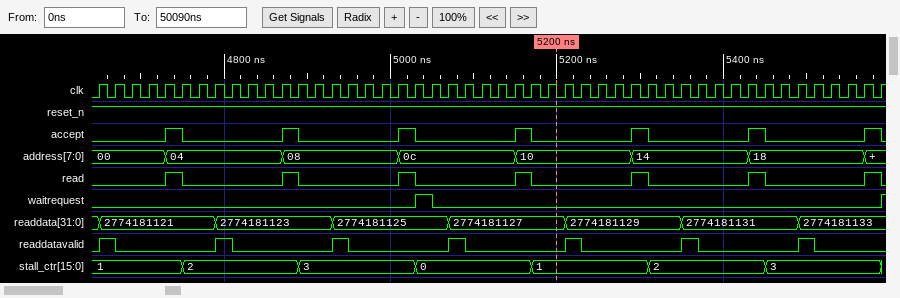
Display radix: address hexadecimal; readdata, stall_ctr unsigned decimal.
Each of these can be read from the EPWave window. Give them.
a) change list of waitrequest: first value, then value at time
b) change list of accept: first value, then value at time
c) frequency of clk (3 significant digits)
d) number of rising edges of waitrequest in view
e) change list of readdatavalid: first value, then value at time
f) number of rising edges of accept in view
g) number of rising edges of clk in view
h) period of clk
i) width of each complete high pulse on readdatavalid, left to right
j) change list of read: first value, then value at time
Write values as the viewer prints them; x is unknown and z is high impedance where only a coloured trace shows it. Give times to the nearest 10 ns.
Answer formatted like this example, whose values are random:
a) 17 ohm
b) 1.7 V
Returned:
a) 0, 1 at 5030 ns, 0 at 5050 ns, 1 at 5590 ns
b) 0, 1 at 4730 ns, 0 at 4750 ns, 1 at 4870 ns, 0 at 4890 ns, 1 at 5010 ns, 0 at 5030 ns, 1 at 5150 ns, 0 at 5170 ns, 1 at 5290 ns, 0 at 5310 ns, 1 at 5430 ns, 0 at 5450 ns, 1 at 5570 ns, 0 at 5590 ns
c) 50.0 MHz
d) 2
e) 0, 1 at 4650 ns, 0 at 4670 ns, 1 at 4790 ns, 0 at 4810 ns, 1 at 4930 ns, 0 at 4950 ns, 1 at 5070 ns, 0 at 5090 ns, 1 at 5210 ns, 0 at 5230 ns, 1 at 5350 ns, 0 at 5370 ns, 1 at 5490 ns, 0 at 5510 ns
f) 7
g) 48
h) 20 ns
i) 20 ns, 20 ns, 20 ns, 20 ns, 20 ns, 20 ns, 20 ns
j) 0, 1 at 4730 ns, 0 at 4750 ns, 1 at 4870 ns, 0 at 4890 ns, 1 at 5010 ns, 0 at 5030 ns, 1 at 5150 ns, 0 at 5170 ns, 1 at 5290 ns, 0 at 5310 ns, 1 at 5430 ns, 0 at 5450 ns, 1 at 5570 ns, 0 at 5590 ns
